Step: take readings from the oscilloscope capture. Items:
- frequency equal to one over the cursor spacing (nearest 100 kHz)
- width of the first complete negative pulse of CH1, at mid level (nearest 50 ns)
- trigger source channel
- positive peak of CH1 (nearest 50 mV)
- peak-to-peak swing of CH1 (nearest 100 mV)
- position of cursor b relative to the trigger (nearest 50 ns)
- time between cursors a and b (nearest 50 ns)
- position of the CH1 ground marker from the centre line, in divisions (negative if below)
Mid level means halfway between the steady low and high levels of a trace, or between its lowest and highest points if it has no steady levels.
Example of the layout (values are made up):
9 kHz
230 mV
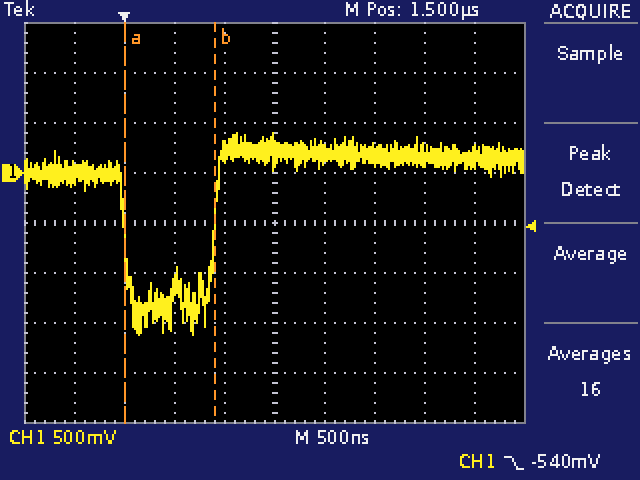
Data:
1.1 MHz
900 ns
CH1
400 mV
2.00 V
+900 ns
900 ns
+1.0 div
